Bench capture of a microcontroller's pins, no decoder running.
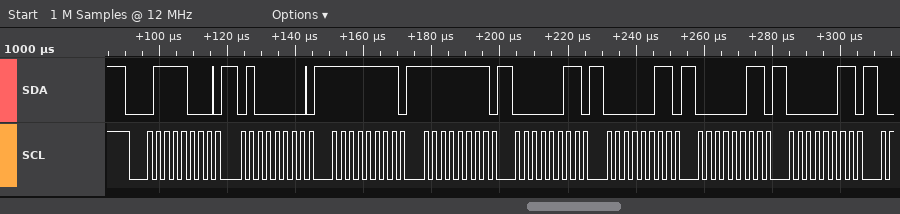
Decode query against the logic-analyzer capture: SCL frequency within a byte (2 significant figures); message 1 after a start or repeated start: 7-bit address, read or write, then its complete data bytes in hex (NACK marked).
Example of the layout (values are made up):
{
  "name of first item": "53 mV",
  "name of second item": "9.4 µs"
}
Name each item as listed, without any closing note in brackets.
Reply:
{
  "SCL frequency within a byte": "400 kHz",
  "message 1 after a start or repeated start: 7-bit address, read or write, then its complete data bytes in hex": "0x3C write: 40 FF FF 03 03 03 03"
}
